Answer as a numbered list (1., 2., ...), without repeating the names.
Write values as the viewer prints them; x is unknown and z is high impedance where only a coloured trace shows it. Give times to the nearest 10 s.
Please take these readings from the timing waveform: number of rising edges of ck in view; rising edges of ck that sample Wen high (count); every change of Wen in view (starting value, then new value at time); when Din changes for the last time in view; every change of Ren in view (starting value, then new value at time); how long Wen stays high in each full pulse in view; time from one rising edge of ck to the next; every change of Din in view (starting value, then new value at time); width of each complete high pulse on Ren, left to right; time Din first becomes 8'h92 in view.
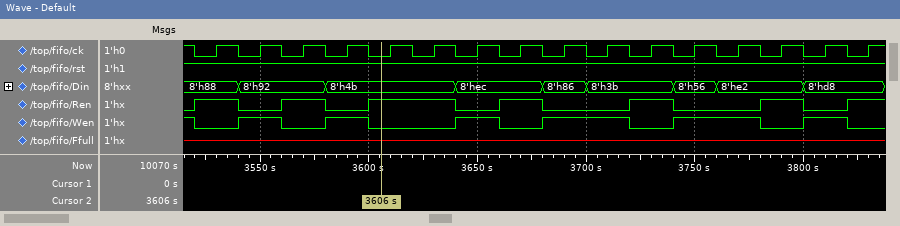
1. 16
2. 8
3. 1, 0 at 3520 s, 1 at 3540 s, 0 at 3560 s, 1 at 3580 s, 0 at 3600 s, 1 at 3640 s, 0 at 3660 s, 1 at 3680 s, 0 at 3720 s, 1 at 3740 s, 0 at 3780 s, 1 at 3800 s, 0 at 3820 s
4. 3800 s
5. 0, 1 at 3520 s, 0 at 3540 s, 1 at 3560 s, 0 at 3580 s, 1 at 3600 s, 0 at 3640 s, 1 at 3660 s, 0 at 3680 s, 1 at 3720 s, 0 at 3740 s, 1 at 3780 s, 0 at 3800 s, 1 at 3820 s
6. 20 s, 20 s, 20 s, 40 s, 40 s, 20 s
7. 20 s
8. 8'h88, 8'h92 at 3540 s, 8'h4b at 3580 s, 8'hec at 3640 s, 8'h86 at 3680 s, 8'h3b at 3700 s, 8'h56 at 3740 s, 8'he2 at 3760 s, 8'hd8 at 3800 s
9. 20 s, 20 s, 40 s, 20 s, 20 s, 20 s
10. 3540 s
